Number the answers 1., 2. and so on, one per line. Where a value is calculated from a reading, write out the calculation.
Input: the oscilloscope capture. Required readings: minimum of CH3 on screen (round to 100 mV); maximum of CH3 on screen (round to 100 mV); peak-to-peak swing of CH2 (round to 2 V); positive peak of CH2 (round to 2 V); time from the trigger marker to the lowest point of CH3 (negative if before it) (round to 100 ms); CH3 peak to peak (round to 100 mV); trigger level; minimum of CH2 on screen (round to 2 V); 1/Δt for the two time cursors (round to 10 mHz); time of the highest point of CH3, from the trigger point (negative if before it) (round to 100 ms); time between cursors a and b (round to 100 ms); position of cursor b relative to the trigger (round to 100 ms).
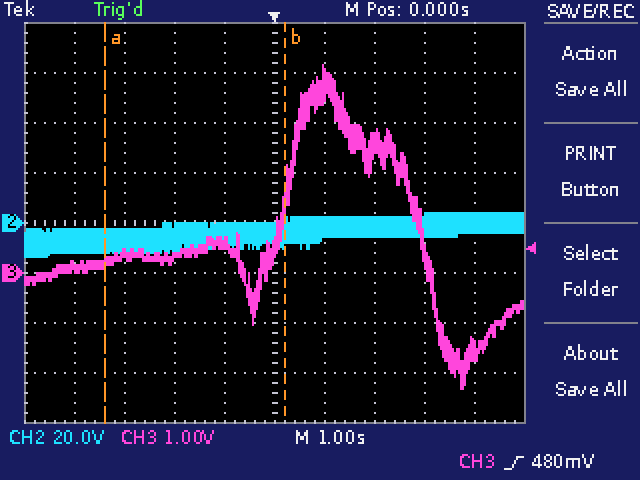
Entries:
1. -2.3 V
2. 4.2 V
3. 4 V − (-14 V) = 18 V
4. 4 V
5. +3.8 s
6. 4.2 V − (-2.3 V) = 6.5 V
7. 480 mV
8. -14 V
9. 1 / 3.6 s ≈ 280 mHz
10. +1.0 s
11. 3.6 s
12. +200 ms
